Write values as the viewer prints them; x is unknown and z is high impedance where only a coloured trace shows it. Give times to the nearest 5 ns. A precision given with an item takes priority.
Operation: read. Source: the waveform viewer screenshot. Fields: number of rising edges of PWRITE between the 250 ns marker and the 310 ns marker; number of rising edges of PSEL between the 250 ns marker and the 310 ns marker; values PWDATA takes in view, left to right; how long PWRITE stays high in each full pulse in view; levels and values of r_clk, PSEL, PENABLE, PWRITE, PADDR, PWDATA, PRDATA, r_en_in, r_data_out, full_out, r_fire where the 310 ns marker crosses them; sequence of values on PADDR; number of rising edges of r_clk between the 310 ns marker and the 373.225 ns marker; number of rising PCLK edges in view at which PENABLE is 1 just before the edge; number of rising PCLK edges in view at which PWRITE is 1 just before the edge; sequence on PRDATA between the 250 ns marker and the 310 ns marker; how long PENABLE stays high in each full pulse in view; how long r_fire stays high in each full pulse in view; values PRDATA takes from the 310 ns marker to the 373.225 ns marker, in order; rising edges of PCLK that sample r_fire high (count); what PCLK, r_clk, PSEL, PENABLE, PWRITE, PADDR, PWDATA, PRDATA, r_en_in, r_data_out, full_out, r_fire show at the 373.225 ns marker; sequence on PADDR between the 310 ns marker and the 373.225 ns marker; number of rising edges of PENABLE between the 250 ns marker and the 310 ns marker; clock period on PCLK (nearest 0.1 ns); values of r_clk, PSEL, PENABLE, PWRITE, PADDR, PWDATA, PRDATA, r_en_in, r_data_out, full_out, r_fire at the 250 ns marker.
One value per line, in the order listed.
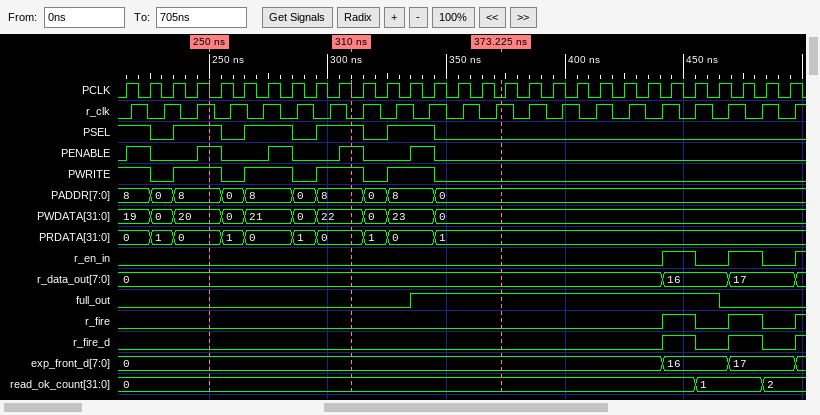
2
2
19, 0, 20, 0, 21, 0, 22, 0, 23, 0
20 ns, 20 ns, 20 ns, 20 ns
r_clk=0, PSEL=1, PENABLE=1, PWRITE=1, PADDR=8, PWDATA=22, PRDATA=0, r_en_in=0, r_data_out=0, full_out=0, r_fire=0
8, 0, 8, 0, 8, 0, 8, 0, 8, 0
5
5
10
0, 1, 0, 1, 0
10 ns, 10 ns, 10 ns, 10 ns, 10 ns
15 ns, 15 ns
0, 1, 0, 1
3
PCLK=0, r_clk=1, PSEL=0, PENABLE=0, PWRITE=0, PADDR=0, PWDATA=0, PRDATA=1, r_en_in=0, r_data_out=0, full_out=1, r_fire=0
8, 0, 8, 0
2
10 ns
r_clk=1, PSEL=1, PENABLE=1, PWRITE=1, PADDR=8, PWDATA=20, PRDATA=0, r_en_in=0, r_data_out=0, full_out=0, r_fire=0
